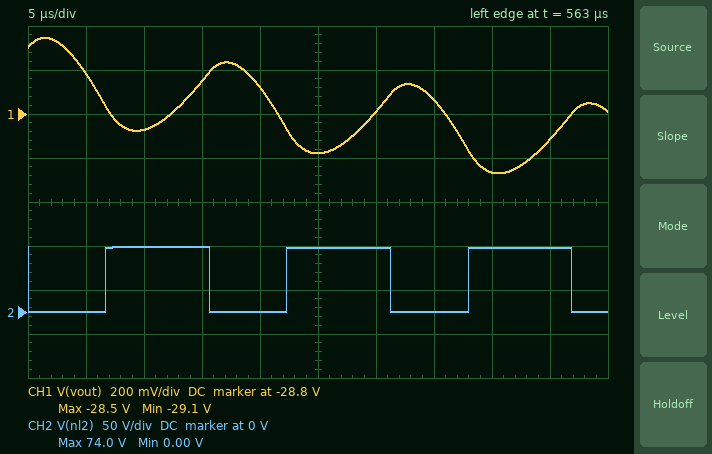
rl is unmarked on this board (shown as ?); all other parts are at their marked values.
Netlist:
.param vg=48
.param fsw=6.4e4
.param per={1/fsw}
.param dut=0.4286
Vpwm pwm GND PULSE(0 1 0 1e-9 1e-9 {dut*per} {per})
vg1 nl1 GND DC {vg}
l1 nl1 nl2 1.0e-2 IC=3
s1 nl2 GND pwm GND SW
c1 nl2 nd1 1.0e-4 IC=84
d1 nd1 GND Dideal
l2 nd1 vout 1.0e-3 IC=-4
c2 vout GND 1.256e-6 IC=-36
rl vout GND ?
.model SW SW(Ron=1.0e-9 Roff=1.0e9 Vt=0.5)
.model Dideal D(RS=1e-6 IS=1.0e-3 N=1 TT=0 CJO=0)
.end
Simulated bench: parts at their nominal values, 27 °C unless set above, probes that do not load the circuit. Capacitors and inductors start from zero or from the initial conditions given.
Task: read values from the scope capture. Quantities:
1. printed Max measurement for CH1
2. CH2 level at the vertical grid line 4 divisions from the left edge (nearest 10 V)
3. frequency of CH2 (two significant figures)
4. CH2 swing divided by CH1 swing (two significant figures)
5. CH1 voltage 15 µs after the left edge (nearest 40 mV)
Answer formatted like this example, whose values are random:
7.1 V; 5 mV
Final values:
-28.5 V; 0 V; 64 kHz; 120; -28.64 V
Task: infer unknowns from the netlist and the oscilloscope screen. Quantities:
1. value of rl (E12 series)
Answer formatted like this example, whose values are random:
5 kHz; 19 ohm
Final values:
2.7 Ω
